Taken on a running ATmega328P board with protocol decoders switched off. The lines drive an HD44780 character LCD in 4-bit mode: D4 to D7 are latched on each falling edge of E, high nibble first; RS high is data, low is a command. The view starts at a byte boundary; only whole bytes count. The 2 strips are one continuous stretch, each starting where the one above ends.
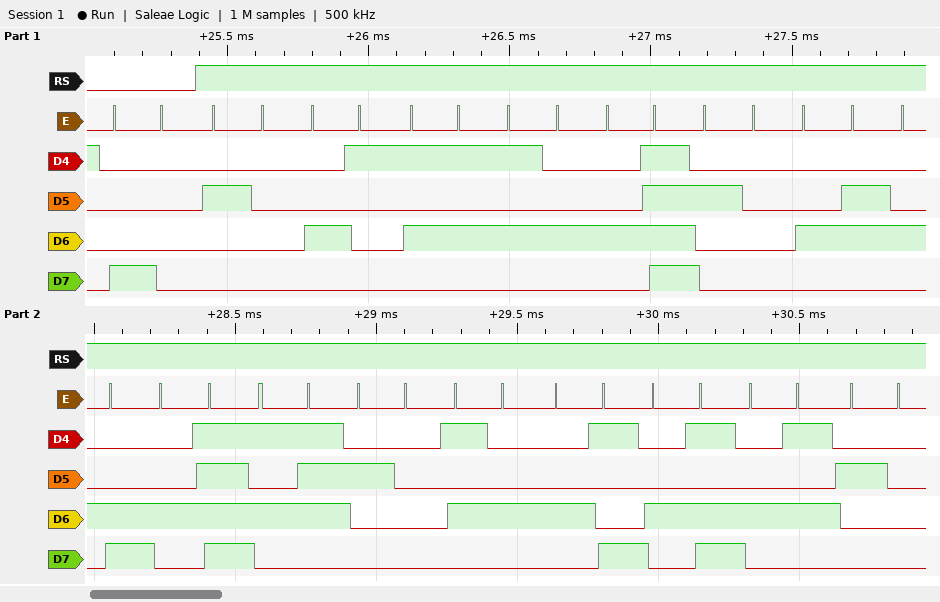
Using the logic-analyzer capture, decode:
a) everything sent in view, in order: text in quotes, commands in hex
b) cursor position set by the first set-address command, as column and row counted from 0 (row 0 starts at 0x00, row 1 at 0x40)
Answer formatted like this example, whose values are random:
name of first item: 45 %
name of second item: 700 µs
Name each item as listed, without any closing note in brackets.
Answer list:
everything sent in view, in order: text in quotes, commands in hex: 0x80 " AUTO FLOW TIME "
cursor position set by the first set-address command, as column and row counted from 0: column 0, row 0
